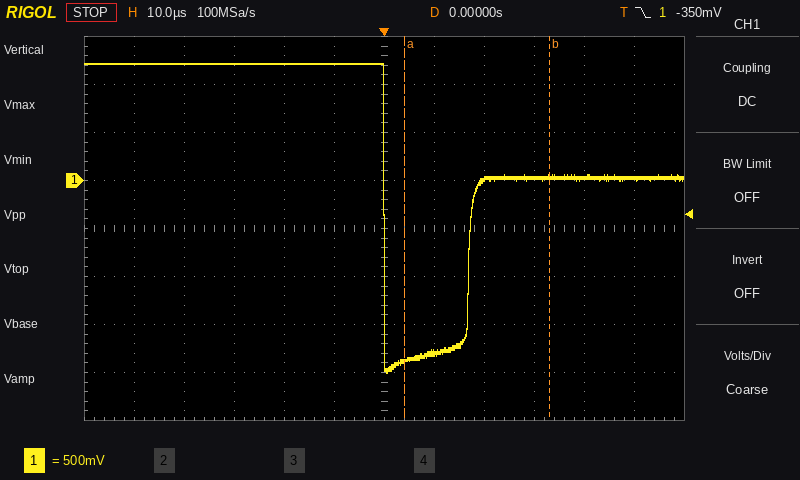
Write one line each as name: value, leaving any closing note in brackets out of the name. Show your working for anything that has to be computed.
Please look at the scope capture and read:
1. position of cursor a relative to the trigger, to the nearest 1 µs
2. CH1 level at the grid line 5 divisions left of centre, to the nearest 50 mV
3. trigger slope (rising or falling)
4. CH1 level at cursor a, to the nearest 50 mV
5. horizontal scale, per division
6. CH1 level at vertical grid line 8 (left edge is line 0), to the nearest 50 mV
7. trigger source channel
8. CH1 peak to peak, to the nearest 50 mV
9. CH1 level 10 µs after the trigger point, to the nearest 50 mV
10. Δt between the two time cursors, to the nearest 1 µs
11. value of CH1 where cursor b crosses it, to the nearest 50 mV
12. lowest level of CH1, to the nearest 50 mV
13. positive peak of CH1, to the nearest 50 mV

position of cursor a relative to the trigger, to the nearest 1 µs: +4 µs
CH1 level at the grid line 5 divisions left of centre, to the nearest 50 mV: 1.20 V
trigger slope: falling
CH1 level at cursor a, to the nearest 50 mV: -1.85 V
horizontal scale, per division: 10 µs
CH1 level at vertical grid line 8 (left edge is line 0), to the nearest 50 mV: 0 mV
trigger source channel: CH1
CH1 peak to peak, to the nearest 50 mV: 1.20 V − (-2.00 V) = 3.20 V
CH1 level 10 µs after the trigger point, to the nearest 50 mV: -1.80 V
Δt between the two time cursors, to the nearest 1 µs: 29 µs
value of CH1 where cursor b crosses it, to the nearest 50 mV: 50 mV
lowest level of CH1, to the nearest 50 mV: -2.00 V
positive peak of CH1, to the nearest 50 mV: 1.20 V
